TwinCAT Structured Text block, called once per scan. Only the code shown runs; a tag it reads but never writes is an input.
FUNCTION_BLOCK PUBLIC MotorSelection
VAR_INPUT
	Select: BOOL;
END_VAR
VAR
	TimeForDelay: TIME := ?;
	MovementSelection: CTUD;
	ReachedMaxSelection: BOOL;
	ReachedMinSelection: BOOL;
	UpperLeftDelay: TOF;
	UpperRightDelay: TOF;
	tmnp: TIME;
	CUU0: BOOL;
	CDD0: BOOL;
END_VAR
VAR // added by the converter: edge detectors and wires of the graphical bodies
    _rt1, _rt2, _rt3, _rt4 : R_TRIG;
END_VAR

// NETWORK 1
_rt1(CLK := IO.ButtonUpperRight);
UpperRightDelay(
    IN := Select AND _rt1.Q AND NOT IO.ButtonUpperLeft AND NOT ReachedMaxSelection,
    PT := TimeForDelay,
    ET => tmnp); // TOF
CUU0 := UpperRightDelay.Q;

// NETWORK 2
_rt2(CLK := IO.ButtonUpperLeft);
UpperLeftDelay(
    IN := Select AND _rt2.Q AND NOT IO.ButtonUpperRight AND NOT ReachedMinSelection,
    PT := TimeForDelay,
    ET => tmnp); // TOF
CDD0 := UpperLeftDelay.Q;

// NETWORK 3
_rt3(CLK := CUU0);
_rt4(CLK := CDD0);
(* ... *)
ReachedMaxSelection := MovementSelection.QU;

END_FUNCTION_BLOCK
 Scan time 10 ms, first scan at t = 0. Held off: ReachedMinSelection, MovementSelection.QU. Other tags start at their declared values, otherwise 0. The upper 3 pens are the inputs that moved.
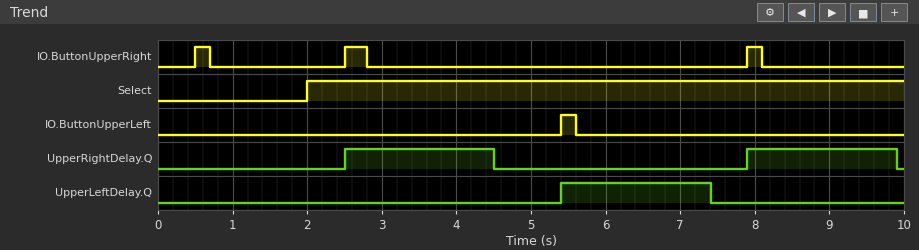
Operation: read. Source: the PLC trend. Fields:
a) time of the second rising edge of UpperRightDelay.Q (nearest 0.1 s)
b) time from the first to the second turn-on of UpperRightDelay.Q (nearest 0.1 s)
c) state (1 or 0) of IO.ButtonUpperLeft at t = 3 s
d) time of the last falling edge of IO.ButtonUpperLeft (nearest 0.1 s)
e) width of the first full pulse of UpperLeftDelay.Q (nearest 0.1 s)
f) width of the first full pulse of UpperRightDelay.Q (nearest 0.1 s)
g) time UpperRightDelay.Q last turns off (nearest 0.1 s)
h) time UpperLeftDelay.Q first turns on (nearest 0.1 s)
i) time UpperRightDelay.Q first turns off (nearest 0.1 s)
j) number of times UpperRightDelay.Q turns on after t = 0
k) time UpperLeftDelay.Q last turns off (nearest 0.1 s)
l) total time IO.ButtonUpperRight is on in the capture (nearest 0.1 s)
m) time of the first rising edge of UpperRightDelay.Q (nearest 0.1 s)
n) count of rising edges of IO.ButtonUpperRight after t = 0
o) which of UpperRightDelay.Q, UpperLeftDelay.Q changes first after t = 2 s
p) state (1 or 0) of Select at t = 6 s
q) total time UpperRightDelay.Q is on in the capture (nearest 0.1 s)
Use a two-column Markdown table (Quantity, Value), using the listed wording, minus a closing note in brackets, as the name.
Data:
| Quantity | Value |
|---|---|
| time of the second rising edge of UpperRightDelay.Q | 7.9 s |
| time from the first to the second turn-on of UpperRightDelay.Q | 5.4 s |
| state (1 or 0) of IO.ButtonUpperLeft at t = 3 s | 0 |
| time of the last falling edge of IO.ButtonUpperLeft | 5.6 s |
| width of the first full pulse of UpperLeftDelay.Q | 2.0 s |
| width of the first full pulse of UpperRightDelay.Q | 2.0 s |
| time UpperRightDelay.Q last turns off | 9.9 s |
| time UpperLeftDelay.Q first turns on | 5.4 s |
| time UpperRightDelay.Q first turns off | 4.5 s |
| number of times UpperRightDelay.Q turns on after t = 0 | 2 |
| time UpperLeftDelay.Q last turns off | 7.4 s |
| total time IO.ButtonUpperRight is on in the capture | 0.7 s |
| time of the first rising edge of UpperRightDelay.Q | 2.5 s |
| count of rising edges of IO.ButtonUpperRight after t = 0 | 3 |
| which of UpperRightDelay.Q, UpperLeftDelay.Q changes first after t = 2 s | UpperRightDelay.Q |
| state (1 or 0) of Select at t = 6 s | 1 |
| total time UpperRightDelay.Q is on in the capture | 4.0 s |
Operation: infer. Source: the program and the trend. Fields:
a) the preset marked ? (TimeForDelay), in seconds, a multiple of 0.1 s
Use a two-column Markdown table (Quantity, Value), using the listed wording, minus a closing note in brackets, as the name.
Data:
| Quantity | Value |
|---|---|
| the preset marked ? (TimeForDelay), in seconds, a multiple of 0.1 s | 2.0 s |
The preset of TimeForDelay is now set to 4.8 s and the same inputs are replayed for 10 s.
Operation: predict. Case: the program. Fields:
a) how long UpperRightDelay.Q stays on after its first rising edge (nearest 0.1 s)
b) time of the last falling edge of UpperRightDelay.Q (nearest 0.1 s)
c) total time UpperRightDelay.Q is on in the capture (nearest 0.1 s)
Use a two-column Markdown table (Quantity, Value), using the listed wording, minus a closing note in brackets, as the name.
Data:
| Quantity | Value |
|---|---|
| how long UpperRightDelay.Q stays on after its first rising edge | 4.8 s |
| time of the last falling edge of UpperRightDelay.Q | 7.3 s |
| total time UpperRightDelay.Q is on in the capture | 6.9 s |
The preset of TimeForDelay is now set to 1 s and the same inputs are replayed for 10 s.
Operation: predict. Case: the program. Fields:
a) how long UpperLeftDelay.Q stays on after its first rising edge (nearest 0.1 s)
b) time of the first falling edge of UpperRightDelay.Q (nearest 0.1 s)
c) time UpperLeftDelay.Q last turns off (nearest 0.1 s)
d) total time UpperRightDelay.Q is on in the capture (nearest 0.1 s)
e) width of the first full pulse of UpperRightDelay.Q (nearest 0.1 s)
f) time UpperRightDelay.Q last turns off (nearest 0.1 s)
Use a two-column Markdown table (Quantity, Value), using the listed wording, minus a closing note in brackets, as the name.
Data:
| Quantity | Value |
|---|---|
| how long UpperLeftDelay.Q stays on after its first rising edge | 1.0 s |
| time of the first falling edge of UpperRightDelay.Q | 3.5 s |
| time UpperLeftDelay.Q last turns off | 6.4 s |
| total time UpperRightDelay.Q is on in the capture | 2.0 s |
| width of the first full pulse of UpperRightDelay.Q | 1.0 s |
| time UpperRightDelay.Q last turns off | 8.9 s |
